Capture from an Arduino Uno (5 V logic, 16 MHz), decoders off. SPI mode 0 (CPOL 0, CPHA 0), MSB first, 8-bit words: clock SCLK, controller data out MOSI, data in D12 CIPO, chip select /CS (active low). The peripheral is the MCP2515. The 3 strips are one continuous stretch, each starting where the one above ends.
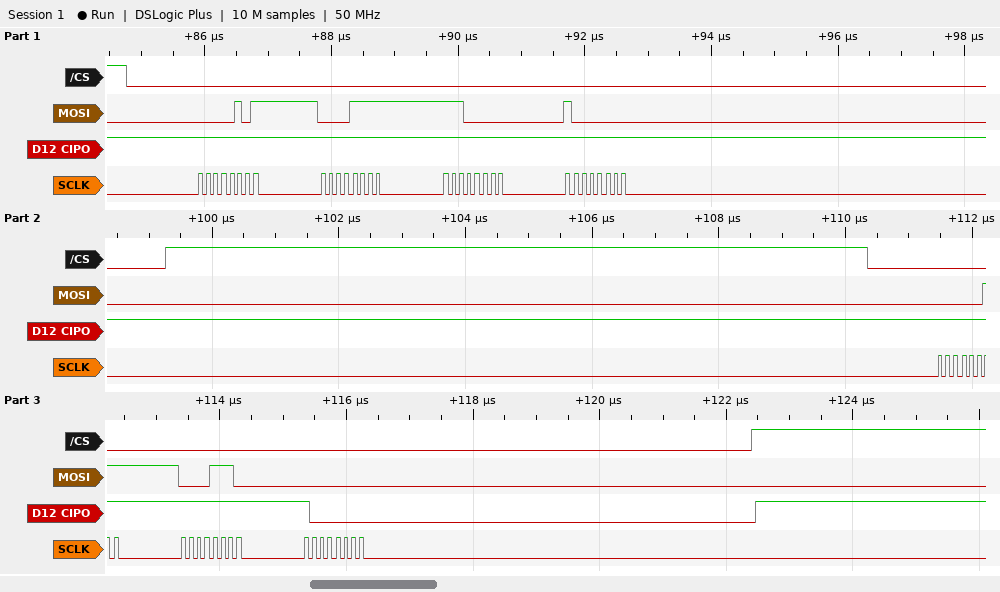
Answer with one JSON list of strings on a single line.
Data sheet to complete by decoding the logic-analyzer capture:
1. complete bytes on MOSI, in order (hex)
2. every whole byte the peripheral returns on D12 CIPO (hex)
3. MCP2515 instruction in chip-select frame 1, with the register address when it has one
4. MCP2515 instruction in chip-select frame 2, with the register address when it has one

["0x05 0x0F 0xE0 0x80 0x03 0x0E 0x00", "0xFF 0xFF 0xFF 0xFF 0xFF 0xFF 0x80", "BIT MODIFY 0x0F", "READ 0x0E"]
